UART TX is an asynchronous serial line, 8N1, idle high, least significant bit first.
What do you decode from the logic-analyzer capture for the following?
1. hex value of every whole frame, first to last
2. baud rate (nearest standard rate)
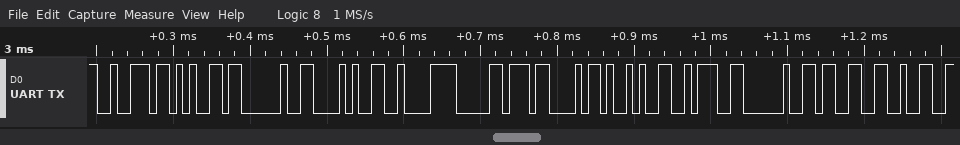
0x72 0x65 0x20 0x28 0xC2 0xB0 0x43 0x29 0x3A 0x20 0x33 0x32
115200 baud
